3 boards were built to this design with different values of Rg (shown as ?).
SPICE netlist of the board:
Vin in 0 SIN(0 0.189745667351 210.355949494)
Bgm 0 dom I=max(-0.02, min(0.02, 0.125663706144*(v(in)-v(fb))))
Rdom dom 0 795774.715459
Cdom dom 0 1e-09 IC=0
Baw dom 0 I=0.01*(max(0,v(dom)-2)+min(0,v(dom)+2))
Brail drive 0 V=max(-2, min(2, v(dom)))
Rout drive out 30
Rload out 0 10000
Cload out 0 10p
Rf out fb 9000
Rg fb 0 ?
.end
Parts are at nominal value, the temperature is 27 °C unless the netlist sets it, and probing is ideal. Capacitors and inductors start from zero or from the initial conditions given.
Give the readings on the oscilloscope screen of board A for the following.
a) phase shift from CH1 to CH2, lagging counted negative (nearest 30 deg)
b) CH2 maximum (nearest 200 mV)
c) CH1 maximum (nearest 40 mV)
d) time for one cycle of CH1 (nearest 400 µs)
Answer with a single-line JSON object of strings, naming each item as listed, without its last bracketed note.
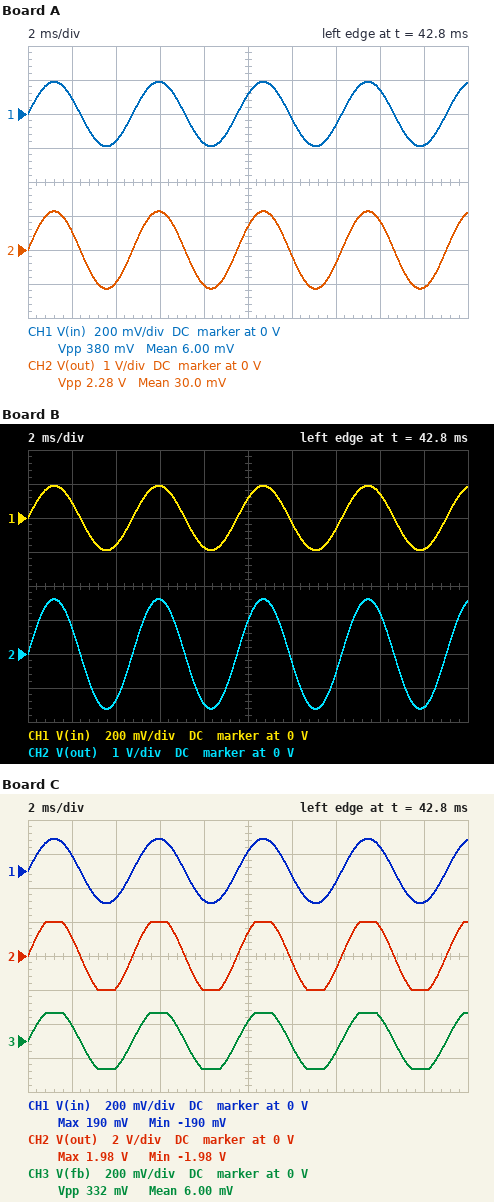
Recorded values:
{"phase shift from CH1 to CH2, lagging counted negative": "0 deg", "CH2 maximum": "1.2 V", "CH1 maximum": "200 mV", "time for one cycle of CH1": "4.8 ms"}
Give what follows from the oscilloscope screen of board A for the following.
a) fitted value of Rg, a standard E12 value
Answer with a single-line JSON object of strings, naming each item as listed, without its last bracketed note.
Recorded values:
{"fitted value of Rg, a standard E12 value": "1.8 kΩ"}
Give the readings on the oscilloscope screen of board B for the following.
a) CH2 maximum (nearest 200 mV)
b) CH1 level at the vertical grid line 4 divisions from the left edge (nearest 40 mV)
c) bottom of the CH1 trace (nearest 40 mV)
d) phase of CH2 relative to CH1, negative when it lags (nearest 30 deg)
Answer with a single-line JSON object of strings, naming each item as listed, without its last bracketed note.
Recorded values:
{"CH2 maximum": "1.6 V", "CH1 level at the vertical grid line 4 divisions from the left edge": "-160 mV", "bottom of the CH1 trace": "-200 mV", "phase of CH2 relative to CH1, negative when it lags": "0 deg"}
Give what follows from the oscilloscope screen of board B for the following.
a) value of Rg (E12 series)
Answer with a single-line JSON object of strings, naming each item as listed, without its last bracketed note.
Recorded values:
{"value of Rg": "1.2 kΩ"}
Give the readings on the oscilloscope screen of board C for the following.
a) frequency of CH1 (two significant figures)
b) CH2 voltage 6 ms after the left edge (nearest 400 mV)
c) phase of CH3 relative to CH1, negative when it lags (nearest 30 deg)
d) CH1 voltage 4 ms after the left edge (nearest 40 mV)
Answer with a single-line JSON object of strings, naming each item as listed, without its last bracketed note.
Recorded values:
{"frequency of CH1": "210 Hz", "CH2 voltage 6 ms after the left edge": "2.0 V", "phase of CH3 relative to CH1, negative when it lags": "0 deg", "CH1 voltage 4 ms after the left edge": "-160 mV"}
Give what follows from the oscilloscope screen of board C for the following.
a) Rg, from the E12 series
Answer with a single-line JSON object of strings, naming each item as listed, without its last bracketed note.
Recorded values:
{"Rg, from the E12 series": "820 Ω"}
